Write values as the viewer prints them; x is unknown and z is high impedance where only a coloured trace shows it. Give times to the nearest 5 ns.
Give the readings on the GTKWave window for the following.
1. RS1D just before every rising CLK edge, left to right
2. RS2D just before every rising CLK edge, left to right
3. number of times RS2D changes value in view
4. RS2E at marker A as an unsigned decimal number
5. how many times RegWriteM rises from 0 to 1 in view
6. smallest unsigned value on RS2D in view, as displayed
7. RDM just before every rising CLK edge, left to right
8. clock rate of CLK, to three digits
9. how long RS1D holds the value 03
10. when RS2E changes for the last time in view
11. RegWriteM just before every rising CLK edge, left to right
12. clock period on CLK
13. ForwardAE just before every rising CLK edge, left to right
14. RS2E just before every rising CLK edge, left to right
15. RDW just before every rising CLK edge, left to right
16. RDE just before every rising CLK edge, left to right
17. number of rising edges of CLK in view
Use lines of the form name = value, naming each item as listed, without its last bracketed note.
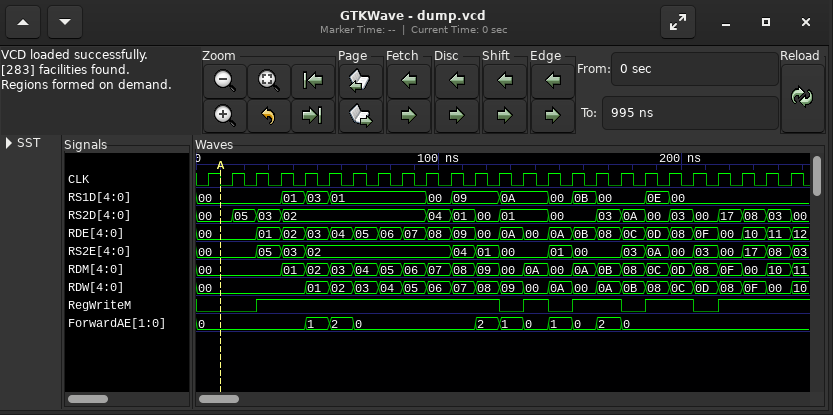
RS1D just before every rising CLK edge, left to right = 00, 00, 00, 00, 01, 03, 01, 01, 01, 01, 00, 09, 09, 0A, 0A, 00, 0B, 00, 00, 0E, 00, 00, 00, 00, 00
RS2D just before every rising CLK edge, left to right = 00, 00, 05, 03, 02, 02, 02, 02, 02, 02, 04, 01, 00, 01, 01, 00, 00, 03, 0A, 00, 03, 00, 17, 08, 03
number of times RS2D changes value in view = 17
RS2E at marker A as an unsigned decimal number = 0
how many times RegWriteM rises from 0 to 1 in view = 5
smallest unsigned value on RS2D in view, as displayed = 00
RDM just before every rising CLK edge, left to right = 00, 00, 00, 00, 01, 02, 03, 04, 05, 06, 07, 08, 09, 00, 0A, 00, 0A, 0B, 08, 0C, 0D, 08, 0F, 00, 10
clock rate of CLK, to three digits = 100 MHz
how long RS1D holds the value 03 = 10 ns
when RS2E changes for the last time in view = 245 ns
RegWriteM just before every rising CLK edge, left to right = 0 0 0 1 1 1 1 1 1 1 1 1 1 0 1 0 1 1 0 1 1 0 1 1 1
clock period on CLK = 10 ns
ForwardAE just before every rising CLK edge, left to right = 0, 0, 0, 0, 0, 1, 2, 0, 0, 0, 0, 0, 2, 1, 0, 1, 0, 2, 0, 0, 0, 0, 0, 0, 0
RS2E just before every rising CLK edge, left to right = 00, 00, 00, 05, 03, 02, 02, 02, 02, 02, 02, 04, 01, 00, 00, 01, 00, 00, 03, 0A, 00, 03, 00, 17, 08
RDW just before every rising CLK edge, left to right = 00, 00, 00, 00, 00, 01, 02, 03, 04, 05, 06, 07, 08, 09, 00, 0A, 00, 0A, 0B, 08, 0C, 0D, 08, 0F, 00
RDE just before every rising CLK edge, left to right = 00, 00, 00, 01, 02, 03, 04, 05, 06, 07, 08, 09, 00, 0A, 00, 0A, 0B, 08, 0C, 0D, 08, 0F, 00, 10, 11
number of rising edges of CLK in view = 25
